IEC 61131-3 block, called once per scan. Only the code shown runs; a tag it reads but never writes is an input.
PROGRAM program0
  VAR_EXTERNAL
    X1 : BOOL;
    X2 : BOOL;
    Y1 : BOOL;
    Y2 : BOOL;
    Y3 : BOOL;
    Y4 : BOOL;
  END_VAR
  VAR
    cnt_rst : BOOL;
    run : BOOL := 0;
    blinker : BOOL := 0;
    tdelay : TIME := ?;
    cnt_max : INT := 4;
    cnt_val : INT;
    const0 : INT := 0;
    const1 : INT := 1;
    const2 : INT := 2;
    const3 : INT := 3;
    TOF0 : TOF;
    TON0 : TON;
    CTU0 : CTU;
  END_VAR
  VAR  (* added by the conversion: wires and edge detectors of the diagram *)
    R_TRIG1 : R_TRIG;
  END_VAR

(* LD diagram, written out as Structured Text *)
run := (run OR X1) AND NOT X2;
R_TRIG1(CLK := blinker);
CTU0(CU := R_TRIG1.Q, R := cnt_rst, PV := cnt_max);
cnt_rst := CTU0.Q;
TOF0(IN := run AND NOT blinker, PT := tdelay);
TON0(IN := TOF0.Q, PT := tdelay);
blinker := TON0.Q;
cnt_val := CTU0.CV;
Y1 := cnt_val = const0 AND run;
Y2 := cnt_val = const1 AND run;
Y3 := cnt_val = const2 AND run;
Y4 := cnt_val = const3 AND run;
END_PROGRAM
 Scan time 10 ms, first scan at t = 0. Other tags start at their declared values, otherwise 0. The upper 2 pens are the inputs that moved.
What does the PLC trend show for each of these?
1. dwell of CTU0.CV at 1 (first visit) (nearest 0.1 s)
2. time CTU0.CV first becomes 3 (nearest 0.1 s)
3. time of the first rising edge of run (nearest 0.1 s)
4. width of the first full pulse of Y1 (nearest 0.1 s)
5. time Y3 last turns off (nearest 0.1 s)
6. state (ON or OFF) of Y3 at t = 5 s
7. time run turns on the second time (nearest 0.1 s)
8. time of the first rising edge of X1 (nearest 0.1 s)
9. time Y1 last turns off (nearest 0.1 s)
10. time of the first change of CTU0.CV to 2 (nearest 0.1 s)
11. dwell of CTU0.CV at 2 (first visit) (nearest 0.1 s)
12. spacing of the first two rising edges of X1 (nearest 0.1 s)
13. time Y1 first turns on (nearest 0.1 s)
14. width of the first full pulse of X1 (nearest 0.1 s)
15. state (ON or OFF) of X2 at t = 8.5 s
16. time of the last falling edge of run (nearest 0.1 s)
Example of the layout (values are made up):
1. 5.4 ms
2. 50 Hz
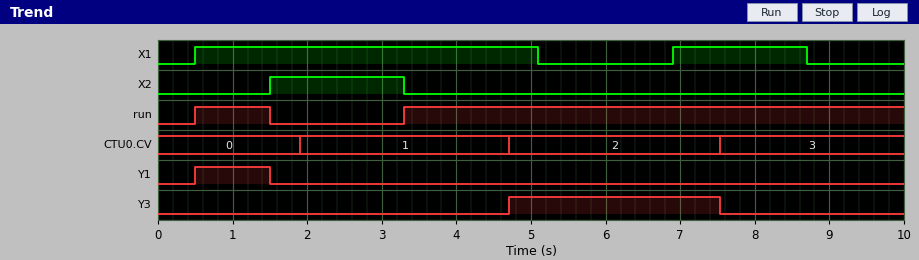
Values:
1. 2.8 s
2. 7.5 s
3. 0.5 s
4. 1.0 s
5. 7.5 s
6. ON
7. 3.3 s
8. 0.5 s
9. 1.5 s
10. 4.7 s
11. 2.8 s
12. 6.4 s
13. 0.5 s
14. 4.6 s
15. OFF
16. 1.5 s
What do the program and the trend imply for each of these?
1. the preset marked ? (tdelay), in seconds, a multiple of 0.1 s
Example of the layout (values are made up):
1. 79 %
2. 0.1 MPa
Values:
1. 1.4 s
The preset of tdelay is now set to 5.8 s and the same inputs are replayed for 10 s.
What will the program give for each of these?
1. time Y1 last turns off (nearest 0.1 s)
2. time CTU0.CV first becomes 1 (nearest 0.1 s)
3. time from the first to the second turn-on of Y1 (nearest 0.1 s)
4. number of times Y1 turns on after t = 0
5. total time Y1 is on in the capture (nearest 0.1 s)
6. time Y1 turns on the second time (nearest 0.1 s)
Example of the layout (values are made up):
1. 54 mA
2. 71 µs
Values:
1. 6.3 s
2. 6.3 s
3. 2.8 s
4. 2
5. 4.0 s
6. 3.3 s
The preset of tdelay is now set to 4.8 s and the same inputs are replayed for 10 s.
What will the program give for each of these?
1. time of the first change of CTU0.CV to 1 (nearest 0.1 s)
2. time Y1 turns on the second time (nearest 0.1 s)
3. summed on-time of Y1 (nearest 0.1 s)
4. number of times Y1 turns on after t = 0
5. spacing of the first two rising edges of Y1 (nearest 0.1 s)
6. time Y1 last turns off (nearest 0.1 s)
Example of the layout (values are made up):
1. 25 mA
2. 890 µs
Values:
1. 5.3 s
2. 3.3 s
3. 3.0 s
4. 2
5. 2.8 s
6. 5.3 s
